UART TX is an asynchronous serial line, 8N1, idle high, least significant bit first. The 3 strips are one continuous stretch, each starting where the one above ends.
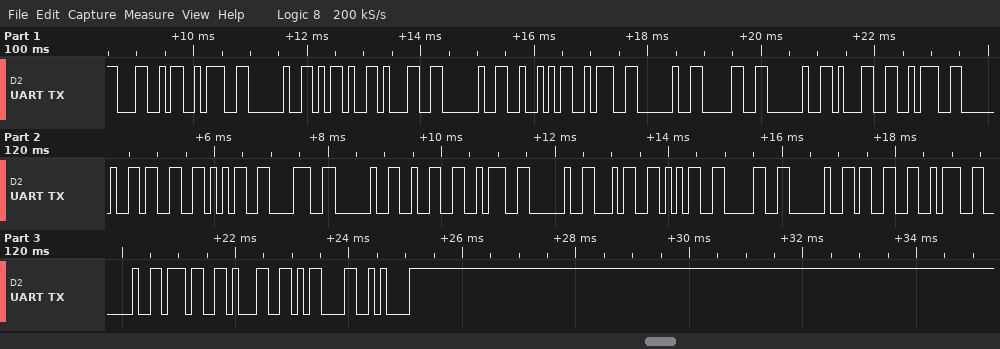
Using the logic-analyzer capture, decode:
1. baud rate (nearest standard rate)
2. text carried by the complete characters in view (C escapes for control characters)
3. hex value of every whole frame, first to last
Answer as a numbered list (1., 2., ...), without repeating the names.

1. 9600 baud
2. "L: -1 R: 0 1: 358 2: 450 3: 71\r\n"
3. 4C 3A 20 2D 31 20 52 3A 20 30 20 31 3A 20 33 35 38 20 32 3A 20 34 35 30 20 33 3A 20 37 31 0D 0A
